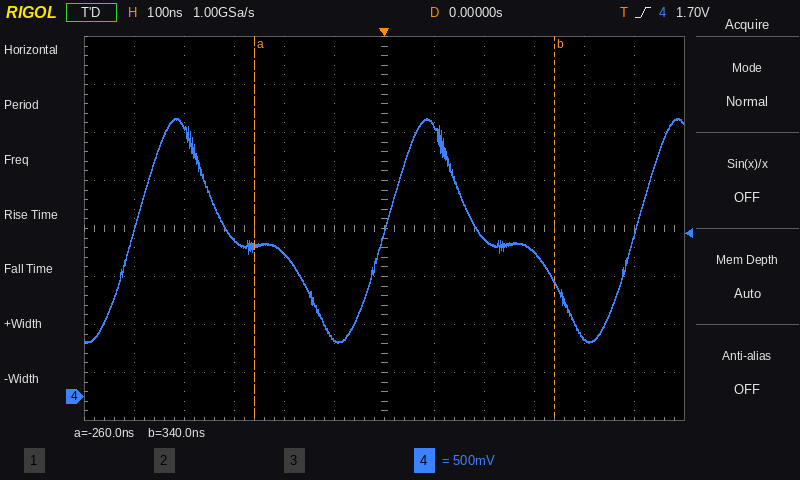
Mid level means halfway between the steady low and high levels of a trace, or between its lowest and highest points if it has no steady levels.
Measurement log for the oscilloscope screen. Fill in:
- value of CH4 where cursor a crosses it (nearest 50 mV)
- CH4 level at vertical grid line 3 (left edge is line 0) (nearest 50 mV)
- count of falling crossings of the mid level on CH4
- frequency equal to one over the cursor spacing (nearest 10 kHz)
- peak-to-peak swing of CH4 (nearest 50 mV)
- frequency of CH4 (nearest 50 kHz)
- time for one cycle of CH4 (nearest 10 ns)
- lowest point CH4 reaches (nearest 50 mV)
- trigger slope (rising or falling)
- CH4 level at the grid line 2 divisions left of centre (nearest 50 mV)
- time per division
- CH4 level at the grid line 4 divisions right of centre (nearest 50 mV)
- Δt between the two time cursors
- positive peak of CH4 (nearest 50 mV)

1.55 V
1.65 V
2
1.67 MHz
2.35 V
2.00 MHz
500 ns
550 mV
rising
1.50 V
100 ns
600 mV
600 ns
2.90 V
